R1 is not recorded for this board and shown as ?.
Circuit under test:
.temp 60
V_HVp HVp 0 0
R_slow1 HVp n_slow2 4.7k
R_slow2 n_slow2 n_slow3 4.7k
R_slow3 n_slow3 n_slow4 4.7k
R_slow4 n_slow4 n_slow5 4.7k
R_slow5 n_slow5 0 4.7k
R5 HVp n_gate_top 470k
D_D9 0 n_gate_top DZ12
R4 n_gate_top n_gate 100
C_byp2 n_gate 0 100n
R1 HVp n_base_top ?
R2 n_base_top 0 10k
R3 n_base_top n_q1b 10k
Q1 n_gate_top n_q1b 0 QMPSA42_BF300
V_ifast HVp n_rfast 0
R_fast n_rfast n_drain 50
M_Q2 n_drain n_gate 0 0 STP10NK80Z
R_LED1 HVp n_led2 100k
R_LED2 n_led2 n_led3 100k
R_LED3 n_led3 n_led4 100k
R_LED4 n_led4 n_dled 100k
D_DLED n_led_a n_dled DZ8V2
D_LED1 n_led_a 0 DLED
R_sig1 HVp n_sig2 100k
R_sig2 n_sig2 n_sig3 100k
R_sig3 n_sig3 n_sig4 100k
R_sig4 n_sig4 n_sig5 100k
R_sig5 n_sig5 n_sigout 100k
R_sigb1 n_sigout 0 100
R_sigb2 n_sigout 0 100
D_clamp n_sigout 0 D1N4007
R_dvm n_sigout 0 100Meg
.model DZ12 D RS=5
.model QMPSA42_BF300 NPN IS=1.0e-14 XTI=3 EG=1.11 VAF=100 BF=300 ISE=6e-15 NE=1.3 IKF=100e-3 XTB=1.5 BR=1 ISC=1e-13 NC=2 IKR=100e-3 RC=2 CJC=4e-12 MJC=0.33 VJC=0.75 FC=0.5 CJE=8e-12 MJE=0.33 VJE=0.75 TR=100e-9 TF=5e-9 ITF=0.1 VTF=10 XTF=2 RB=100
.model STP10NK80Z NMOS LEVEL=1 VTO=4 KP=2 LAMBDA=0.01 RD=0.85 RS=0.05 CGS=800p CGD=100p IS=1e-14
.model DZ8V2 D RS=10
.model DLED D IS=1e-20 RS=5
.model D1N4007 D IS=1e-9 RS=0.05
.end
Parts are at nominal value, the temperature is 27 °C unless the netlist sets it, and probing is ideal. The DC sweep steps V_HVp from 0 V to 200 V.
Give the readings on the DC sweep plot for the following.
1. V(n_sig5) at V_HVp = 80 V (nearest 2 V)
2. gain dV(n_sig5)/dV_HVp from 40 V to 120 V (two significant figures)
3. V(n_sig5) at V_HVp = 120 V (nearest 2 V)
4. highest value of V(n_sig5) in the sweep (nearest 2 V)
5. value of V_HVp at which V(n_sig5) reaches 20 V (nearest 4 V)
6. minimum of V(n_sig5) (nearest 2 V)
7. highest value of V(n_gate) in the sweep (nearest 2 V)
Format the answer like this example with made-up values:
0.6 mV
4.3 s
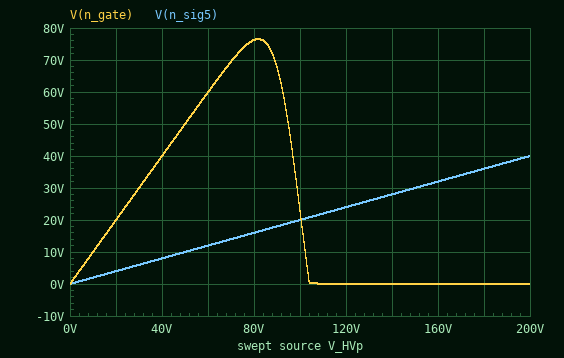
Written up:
16 V
0.20 V/V
24 V
40 V
100 V
0 V
76 V
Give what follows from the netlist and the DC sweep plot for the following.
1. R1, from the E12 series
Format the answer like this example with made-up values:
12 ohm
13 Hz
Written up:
1.8 MΩ
